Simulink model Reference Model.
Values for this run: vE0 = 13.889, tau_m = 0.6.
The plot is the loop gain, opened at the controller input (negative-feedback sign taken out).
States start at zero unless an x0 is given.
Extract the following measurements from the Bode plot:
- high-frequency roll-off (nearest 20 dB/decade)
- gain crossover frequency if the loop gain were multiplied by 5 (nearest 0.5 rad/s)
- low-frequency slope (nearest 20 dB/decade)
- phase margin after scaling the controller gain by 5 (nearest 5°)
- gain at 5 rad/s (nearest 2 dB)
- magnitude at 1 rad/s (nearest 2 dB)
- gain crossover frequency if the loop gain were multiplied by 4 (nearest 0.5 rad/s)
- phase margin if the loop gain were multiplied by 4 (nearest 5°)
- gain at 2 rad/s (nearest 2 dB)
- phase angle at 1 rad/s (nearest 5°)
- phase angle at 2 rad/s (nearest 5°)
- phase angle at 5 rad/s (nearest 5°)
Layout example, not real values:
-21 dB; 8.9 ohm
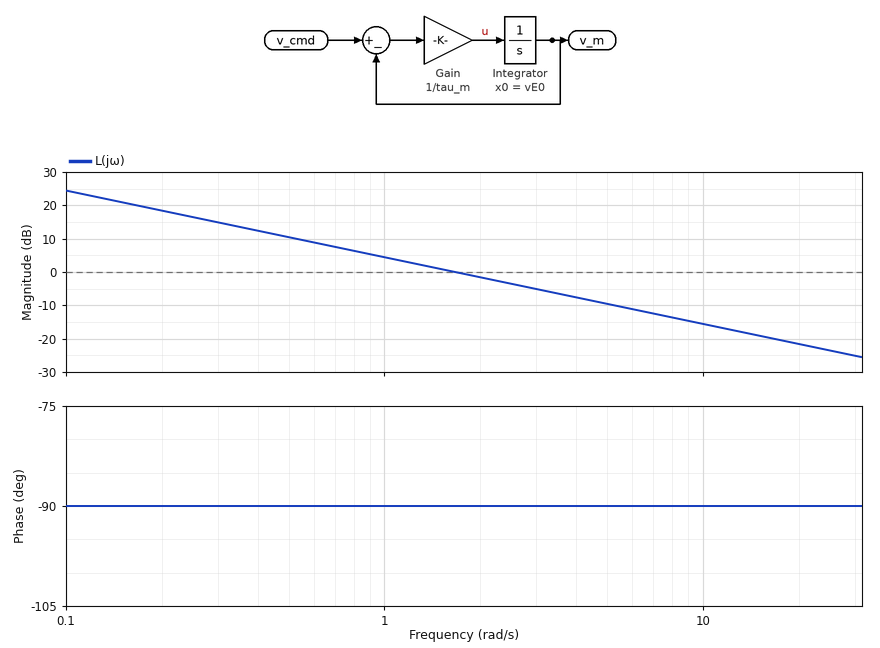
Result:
-20 dB/decade; 8.5 rad/s; -20 dB/decade; 90°; -10 dB; 4 dB; 6.5 rad/s; 90°; -2 dB; -90°; -90°; -90°
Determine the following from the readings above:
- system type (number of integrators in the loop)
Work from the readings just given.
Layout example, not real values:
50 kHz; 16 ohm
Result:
1
